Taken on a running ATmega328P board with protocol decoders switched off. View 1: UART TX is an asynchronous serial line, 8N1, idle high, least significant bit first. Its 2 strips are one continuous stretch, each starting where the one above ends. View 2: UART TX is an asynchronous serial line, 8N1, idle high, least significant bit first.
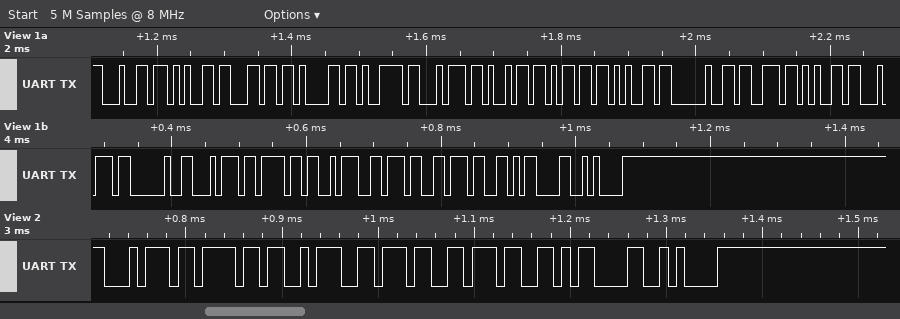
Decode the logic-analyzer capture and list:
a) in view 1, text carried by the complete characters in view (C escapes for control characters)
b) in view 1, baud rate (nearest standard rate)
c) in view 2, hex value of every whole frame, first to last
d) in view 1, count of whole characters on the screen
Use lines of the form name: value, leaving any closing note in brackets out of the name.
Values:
in view 1, text carried by the complete characters in view: "delaytime set to:77\r\n"
in view 1, baud rate: 115200 baud
in view 2, hex value of every whole frame, first to last: 74 6F 3A 37 37 0D 0A
in view 1, count of whole characters on the screen: 21
